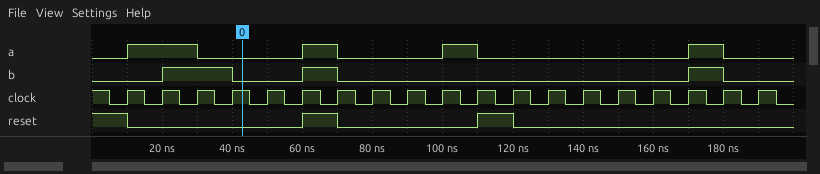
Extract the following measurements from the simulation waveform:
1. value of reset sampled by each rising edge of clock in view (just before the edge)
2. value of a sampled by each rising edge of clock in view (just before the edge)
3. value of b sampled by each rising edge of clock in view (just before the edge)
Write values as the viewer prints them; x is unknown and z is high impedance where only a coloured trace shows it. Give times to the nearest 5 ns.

1 0 0 0 0 0 1 0 0 0 0 1 0 0 0 0 0 0 0
0 1 1 0 0 0 1 0 0 0 1 0 0 0 0 0 0 1 0
0 0 1 1 0 0 1 0 0 0 0 0 0 0 0 0 0 1 0
